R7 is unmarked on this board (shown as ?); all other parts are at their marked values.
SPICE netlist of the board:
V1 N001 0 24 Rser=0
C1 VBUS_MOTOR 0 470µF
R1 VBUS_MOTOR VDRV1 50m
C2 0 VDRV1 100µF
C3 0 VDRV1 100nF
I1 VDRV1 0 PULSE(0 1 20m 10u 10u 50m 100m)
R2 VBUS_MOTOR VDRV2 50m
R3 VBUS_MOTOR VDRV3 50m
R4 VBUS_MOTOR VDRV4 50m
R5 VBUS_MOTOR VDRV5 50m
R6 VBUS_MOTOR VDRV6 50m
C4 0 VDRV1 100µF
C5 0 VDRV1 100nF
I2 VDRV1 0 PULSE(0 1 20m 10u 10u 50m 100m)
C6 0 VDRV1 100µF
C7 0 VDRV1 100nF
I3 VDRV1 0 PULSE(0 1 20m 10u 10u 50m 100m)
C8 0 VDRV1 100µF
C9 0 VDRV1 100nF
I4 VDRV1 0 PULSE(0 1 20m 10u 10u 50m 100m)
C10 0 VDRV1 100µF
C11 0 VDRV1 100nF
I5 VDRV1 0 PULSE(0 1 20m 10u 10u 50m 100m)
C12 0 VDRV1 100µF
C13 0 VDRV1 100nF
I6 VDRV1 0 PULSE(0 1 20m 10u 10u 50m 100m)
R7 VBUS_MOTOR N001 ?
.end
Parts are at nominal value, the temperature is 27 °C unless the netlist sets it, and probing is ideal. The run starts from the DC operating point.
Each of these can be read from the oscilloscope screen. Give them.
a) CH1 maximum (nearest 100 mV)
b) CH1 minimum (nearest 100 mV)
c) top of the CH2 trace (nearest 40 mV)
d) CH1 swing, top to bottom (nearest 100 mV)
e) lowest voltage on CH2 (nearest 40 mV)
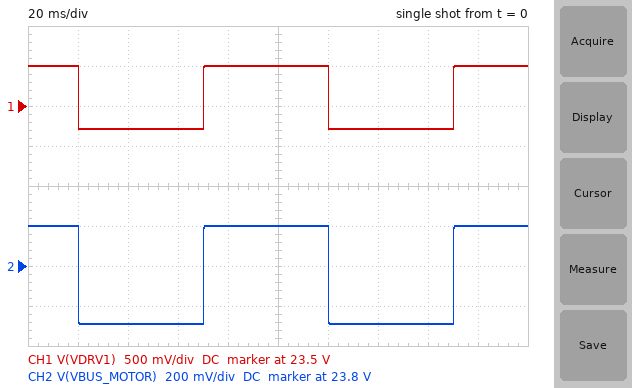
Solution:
24.0 V
23.2 V
24.00 V
800 mV
23.52 V
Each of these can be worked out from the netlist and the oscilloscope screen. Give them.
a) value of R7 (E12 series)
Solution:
0.082 Ω
